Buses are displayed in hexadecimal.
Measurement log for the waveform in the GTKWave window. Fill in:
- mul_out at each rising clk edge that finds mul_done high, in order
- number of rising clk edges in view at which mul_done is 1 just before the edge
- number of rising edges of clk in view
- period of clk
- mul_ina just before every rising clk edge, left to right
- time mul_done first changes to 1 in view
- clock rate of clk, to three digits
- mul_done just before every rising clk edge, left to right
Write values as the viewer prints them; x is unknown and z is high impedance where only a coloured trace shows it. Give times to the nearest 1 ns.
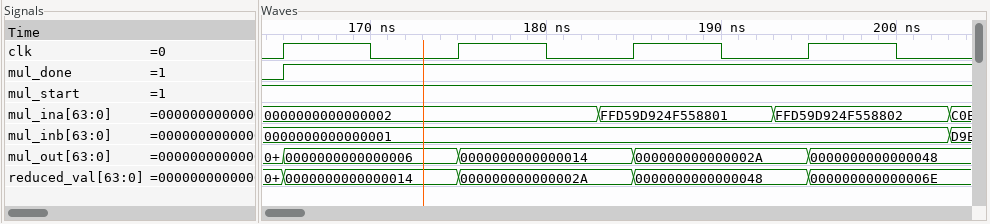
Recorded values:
0000000000000006, 0000000000000014, 000000000000002A
3
4
10 ns
0000000000000002, 0000000000000002, FFD59D924F558801, FFD59D924F558802
165 ns
100 MHz
0 1 1 1
